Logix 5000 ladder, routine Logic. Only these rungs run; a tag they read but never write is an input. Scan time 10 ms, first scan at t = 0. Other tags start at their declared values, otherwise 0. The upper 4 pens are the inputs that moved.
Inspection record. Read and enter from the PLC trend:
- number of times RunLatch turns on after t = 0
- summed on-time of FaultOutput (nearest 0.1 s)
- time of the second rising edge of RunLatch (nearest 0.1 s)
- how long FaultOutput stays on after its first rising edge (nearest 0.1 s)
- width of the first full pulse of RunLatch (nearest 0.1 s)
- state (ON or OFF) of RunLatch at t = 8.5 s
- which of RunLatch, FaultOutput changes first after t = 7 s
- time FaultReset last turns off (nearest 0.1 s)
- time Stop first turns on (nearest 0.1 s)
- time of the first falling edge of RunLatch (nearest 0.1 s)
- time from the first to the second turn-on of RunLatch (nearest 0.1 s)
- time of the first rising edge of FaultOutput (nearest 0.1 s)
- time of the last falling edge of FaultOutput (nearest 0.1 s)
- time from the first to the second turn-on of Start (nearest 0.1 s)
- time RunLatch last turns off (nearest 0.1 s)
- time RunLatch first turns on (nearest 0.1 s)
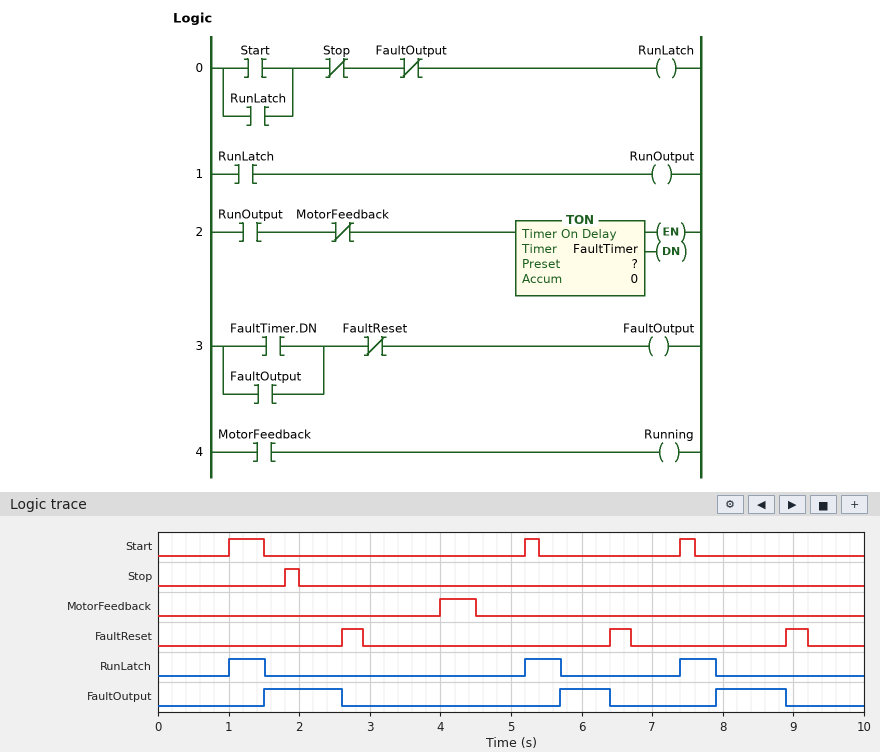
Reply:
3
2.8 s
5.2 s
1.1 s
0.5 s
OFF
RunLatch
9.2 s
1.8 s
1.5 s
4.2 s
1.5 s
8.9 s
4.2 s
7.9 s
1.0 s
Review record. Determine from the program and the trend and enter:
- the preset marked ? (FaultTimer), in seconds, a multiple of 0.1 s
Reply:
0.5 s
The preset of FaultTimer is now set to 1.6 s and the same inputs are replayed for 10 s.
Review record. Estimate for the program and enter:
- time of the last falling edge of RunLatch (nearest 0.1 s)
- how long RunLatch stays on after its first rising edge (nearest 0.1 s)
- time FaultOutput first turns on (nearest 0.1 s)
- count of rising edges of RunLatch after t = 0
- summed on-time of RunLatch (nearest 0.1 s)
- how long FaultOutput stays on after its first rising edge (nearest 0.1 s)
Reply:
6.8 s
0.8 s
6.8 s
2
2.4 s
2.1 s
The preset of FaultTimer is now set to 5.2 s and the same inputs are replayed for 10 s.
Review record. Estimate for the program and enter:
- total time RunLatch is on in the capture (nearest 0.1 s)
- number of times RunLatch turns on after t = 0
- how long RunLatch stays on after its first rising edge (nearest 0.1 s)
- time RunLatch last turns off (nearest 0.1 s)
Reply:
5.6 s
2
0.8 s
1.8 s
